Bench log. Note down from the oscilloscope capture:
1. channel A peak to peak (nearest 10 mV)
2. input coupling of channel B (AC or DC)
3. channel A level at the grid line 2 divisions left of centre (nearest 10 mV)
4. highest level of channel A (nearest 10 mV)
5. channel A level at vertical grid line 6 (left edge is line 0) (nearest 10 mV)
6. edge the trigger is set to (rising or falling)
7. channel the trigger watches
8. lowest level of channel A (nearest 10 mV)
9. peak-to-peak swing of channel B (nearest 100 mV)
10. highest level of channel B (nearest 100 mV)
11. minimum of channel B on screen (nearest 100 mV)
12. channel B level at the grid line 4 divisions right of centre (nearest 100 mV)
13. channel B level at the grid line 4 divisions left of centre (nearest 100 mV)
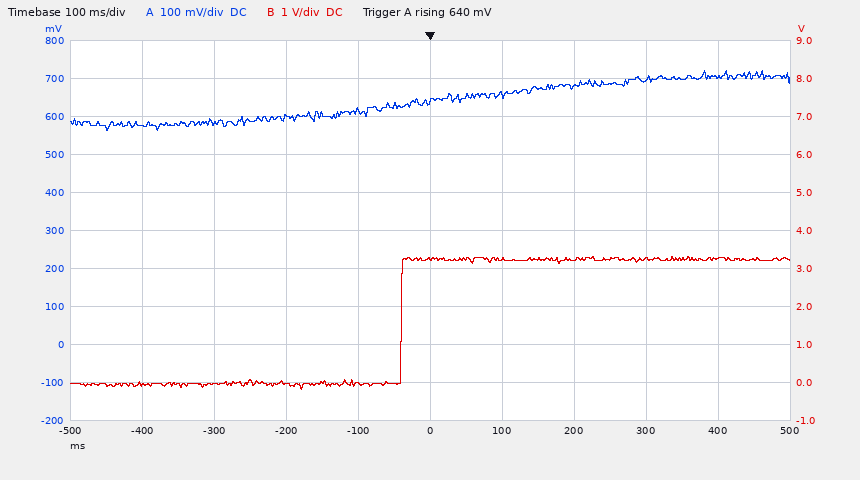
160 mV
DC
600 mV
720 mV
660 mV
rising
channel A
560 mV
3.5 V
3.3 V
-200 mV
3.3 V
0.0 V
